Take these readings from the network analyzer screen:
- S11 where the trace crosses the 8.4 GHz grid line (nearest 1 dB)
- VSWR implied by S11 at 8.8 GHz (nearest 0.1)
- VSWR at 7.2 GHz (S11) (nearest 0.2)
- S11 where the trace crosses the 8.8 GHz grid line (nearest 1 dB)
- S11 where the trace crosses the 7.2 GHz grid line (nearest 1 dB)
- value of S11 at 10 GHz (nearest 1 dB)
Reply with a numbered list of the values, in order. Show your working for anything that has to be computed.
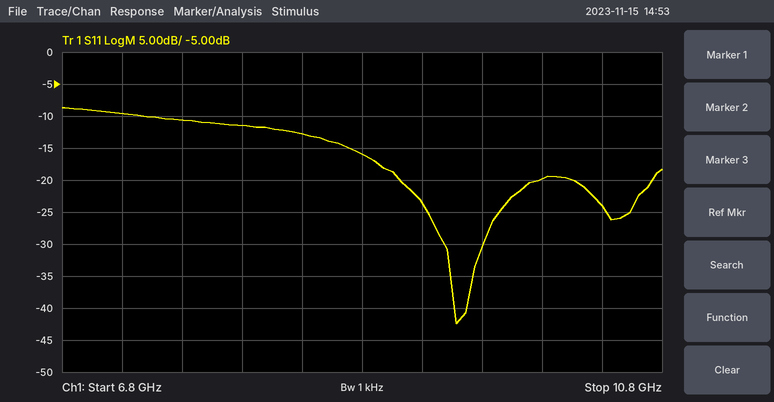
1. -13 dB
2. |Γ| = 10^(-16/20) = 0.1585; VSWR = (1 + 0.1585)/(1 − 0.1585) ≈ 1.4
3. |Γ| = 10^(-10/20) = 0.3162; VSWR = (1 + 0.3162)/(1 − 0.3162) ≈ 1.92, so 2.0 to the nearest 0.2
4. -16 dB
5. -10 dB
6. -20 dB
